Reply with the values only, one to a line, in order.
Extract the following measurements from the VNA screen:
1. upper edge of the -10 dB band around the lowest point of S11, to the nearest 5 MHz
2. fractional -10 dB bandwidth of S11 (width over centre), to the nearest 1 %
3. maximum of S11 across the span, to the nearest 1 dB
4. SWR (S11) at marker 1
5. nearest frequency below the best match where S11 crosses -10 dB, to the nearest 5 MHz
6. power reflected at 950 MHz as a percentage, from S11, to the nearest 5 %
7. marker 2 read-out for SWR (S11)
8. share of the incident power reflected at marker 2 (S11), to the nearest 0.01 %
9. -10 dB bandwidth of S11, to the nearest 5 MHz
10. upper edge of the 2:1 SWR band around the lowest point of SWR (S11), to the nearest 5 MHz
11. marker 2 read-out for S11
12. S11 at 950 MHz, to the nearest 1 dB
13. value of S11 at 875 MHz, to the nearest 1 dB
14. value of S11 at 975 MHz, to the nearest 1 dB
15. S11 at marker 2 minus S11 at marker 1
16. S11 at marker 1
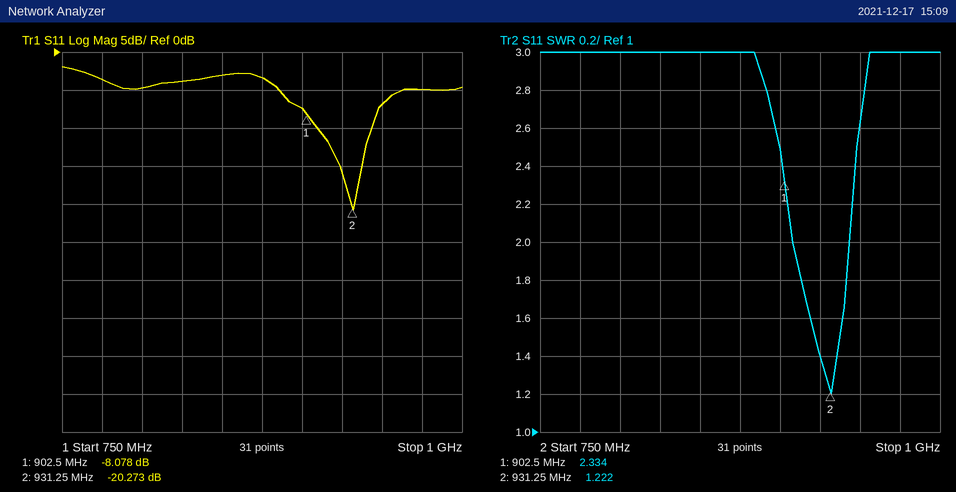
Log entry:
945 MHz
4 %
-2 dB
2.334
910 MHz
20 %
1.222
0.94 %
35 MHz
945 MHz
-20.273 dB
-7 dB
-3 dB
-5 dB
-12.195 dB
-8.078 dB
